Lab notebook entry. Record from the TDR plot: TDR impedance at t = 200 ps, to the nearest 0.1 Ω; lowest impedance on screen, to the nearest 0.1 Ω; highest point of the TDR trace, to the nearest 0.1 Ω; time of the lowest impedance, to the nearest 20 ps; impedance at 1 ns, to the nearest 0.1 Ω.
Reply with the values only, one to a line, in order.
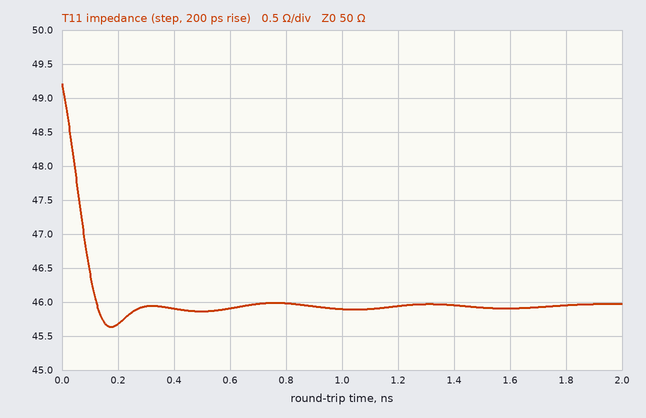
45.7 Ω
45.6 Ω
49.2 Ω
180 ps
45.9 Ω
